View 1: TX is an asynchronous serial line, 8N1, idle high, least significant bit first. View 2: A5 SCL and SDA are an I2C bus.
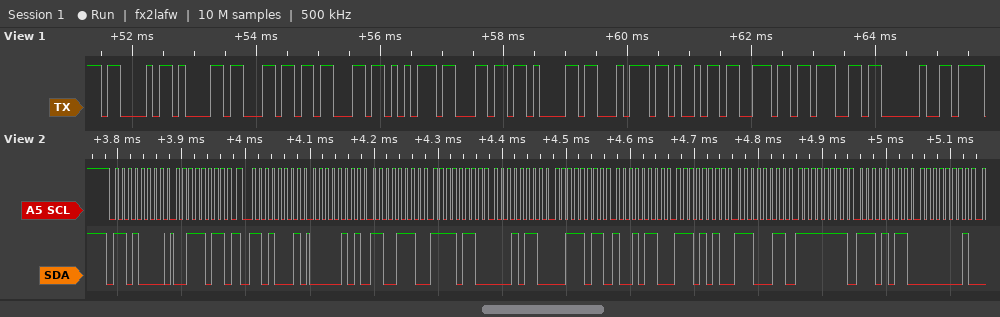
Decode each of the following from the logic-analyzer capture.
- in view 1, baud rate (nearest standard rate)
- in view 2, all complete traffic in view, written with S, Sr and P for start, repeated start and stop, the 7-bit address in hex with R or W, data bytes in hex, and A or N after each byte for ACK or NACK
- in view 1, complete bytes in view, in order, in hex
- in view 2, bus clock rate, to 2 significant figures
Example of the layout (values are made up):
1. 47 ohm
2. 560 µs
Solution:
1. 9600 baud
2. S 68W A 3B A Sr 68R A 05 A CE A F6 A 16 A 3B A 96 A EA A E3 A FF A EB A 01 A
3. 43 61 6C 63 75 6C 61 74 69 6E 67 20
4. 100 kHz
